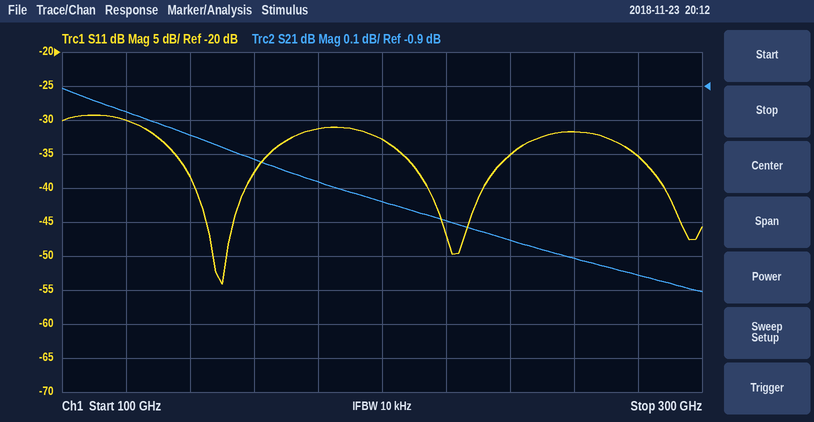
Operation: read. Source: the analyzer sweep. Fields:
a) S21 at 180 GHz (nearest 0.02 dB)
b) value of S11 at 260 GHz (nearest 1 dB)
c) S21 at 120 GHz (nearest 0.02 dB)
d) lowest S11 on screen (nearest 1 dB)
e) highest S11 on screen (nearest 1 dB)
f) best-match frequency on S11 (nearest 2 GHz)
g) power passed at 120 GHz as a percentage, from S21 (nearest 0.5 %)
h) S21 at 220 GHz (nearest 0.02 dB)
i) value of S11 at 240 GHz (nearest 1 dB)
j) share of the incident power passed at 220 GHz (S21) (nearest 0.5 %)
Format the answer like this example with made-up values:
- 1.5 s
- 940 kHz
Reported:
- -1.18 dB
- -32 dB
- -0.98 dB
- -54 dB
- -29 dB
- 150 GHz
- 80.0 %
- -1.30 dB
- -35 dB
- 74.0 %
